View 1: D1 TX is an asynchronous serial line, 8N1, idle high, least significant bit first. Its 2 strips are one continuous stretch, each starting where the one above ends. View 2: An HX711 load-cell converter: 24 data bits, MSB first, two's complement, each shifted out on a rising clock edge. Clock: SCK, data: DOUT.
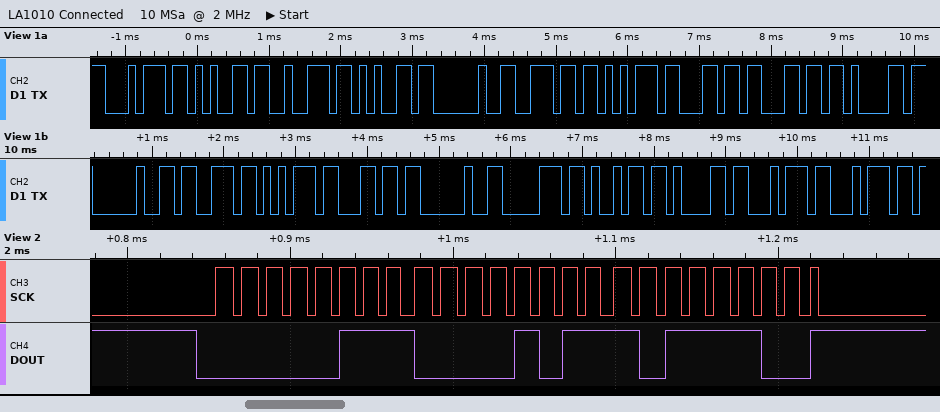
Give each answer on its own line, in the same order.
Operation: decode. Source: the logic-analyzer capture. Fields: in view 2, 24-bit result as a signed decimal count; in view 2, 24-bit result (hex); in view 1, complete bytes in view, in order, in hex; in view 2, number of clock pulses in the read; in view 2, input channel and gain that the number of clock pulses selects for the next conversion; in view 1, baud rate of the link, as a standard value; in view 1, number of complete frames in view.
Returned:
461756
0x070BBC
0x74 0x65 0x72 0x65 0x20 0x6E 0x75 0x6C 0x6C 0x61 0x20 0x73 0x75 0x6C 0x20 0x70 0x69 0x61 0x74 0x74
25
channel A, gain 128
9600 baud
20
